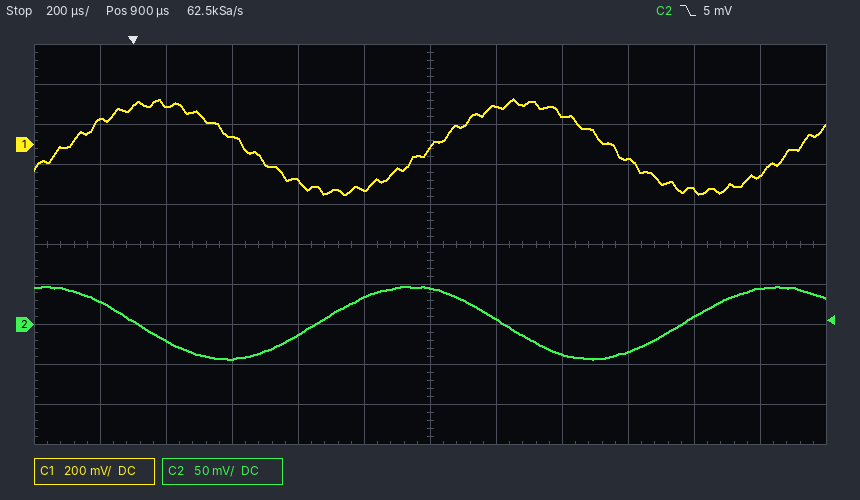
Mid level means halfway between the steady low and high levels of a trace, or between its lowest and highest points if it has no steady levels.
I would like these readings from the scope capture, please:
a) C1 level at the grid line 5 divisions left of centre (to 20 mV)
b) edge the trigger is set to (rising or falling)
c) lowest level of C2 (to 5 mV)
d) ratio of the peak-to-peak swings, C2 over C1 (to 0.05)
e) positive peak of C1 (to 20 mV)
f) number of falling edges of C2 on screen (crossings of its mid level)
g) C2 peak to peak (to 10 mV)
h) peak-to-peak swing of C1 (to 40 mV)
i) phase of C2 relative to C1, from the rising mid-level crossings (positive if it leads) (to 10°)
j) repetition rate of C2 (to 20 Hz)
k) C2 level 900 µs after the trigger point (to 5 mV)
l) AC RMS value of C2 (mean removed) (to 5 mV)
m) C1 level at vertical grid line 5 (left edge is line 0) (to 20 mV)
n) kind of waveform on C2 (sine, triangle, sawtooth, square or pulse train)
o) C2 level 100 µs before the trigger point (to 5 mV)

120 mV
falling
-45 mV
0.20
220 mV
2
90 mV
480 mV
+110°
900 Hz
45 mV
30 mV
-220 mV
sine
30 mV
